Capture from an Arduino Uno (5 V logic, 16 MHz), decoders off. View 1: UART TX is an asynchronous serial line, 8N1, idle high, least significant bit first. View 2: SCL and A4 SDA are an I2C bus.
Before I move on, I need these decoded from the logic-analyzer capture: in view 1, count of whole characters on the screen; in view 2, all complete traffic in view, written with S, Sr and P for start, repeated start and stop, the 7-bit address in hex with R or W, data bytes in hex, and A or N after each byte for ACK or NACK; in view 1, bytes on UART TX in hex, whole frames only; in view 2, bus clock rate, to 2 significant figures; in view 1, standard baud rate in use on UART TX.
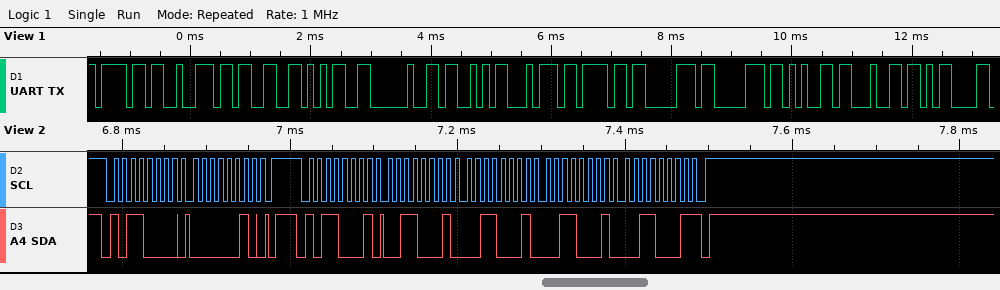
13
S 58W A 02 A P S 58R A 31 A 31 A 31 A 31 N P
6F 72 33 35 20 53 74 6F 70 70 65 64 0D
100 kHz
9600 baud
